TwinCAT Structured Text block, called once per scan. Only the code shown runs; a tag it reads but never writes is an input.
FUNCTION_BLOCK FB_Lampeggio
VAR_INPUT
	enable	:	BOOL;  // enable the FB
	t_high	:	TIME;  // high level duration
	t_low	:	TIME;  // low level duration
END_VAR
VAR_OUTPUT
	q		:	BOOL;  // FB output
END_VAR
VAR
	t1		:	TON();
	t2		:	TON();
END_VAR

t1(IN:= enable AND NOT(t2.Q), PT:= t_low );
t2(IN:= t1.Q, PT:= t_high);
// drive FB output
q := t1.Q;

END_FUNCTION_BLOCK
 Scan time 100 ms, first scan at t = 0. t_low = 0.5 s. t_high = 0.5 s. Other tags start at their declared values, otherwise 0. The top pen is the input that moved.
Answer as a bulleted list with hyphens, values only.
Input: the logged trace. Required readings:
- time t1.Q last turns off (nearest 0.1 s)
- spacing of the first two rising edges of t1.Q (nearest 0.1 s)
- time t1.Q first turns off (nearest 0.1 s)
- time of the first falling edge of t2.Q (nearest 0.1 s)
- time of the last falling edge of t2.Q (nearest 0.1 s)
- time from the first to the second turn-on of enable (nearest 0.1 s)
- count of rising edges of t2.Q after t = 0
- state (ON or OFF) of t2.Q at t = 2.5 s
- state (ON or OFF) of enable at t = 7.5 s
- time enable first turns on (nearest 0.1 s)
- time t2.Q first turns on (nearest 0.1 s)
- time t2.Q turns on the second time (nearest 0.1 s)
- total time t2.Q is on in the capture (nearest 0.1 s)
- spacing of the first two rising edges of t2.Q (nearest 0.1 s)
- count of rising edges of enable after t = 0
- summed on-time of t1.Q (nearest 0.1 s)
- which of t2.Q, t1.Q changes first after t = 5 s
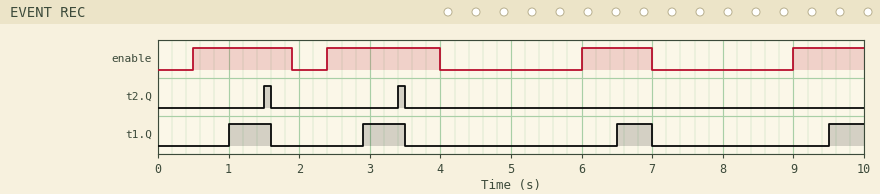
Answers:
- 7.0 s
- 1.9 s
- 1.6 s
- 1.6 s
- 3.5 s
- 1.9 s
- 2
- OFF
- OFF
- 0.5 s
- 1.5 s
- 3.4 s
- 0.2 s
- 1.9 s
- 4
- 2.2 s
- t1.Q
